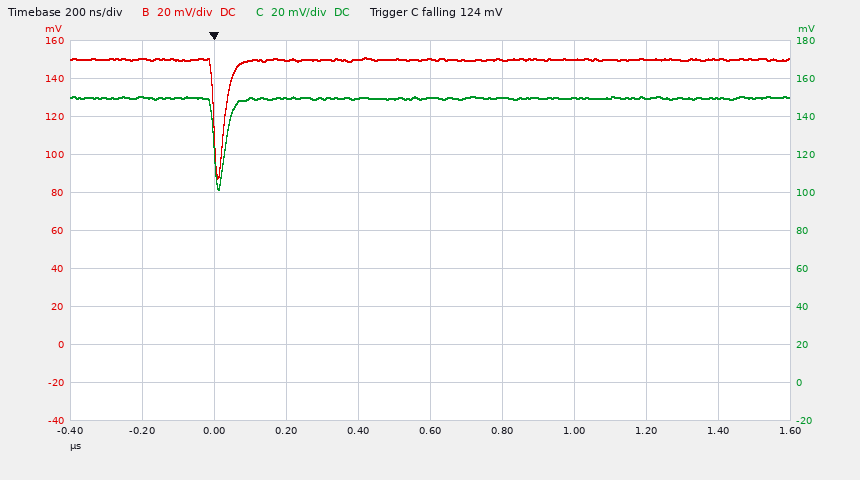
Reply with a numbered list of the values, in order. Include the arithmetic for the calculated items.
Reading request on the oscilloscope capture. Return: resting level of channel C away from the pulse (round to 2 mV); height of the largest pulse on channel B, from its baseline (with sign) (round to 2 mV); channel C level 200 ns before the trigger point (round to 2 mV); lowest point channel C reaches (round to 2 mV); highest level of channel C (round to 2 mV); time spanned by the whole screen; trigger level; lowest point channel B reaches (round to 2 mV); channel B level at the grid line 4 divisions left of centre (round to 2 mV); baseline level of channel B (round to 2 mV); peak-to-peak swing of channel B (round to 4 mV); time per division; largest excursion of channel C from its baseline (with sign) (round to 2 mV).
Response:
1. 150 mV
2. 88 mV − (150 mV) = -62 mV
3. 150 mV
4. 102 mV
5. 150 mV
6. 2 µs
7. 124 mV
8. 88 mV
9. 150 mV
10. 150 mV
11. 64 mV
12. 200 ns
13. 102 mV − (150 mV) = -48 mV
